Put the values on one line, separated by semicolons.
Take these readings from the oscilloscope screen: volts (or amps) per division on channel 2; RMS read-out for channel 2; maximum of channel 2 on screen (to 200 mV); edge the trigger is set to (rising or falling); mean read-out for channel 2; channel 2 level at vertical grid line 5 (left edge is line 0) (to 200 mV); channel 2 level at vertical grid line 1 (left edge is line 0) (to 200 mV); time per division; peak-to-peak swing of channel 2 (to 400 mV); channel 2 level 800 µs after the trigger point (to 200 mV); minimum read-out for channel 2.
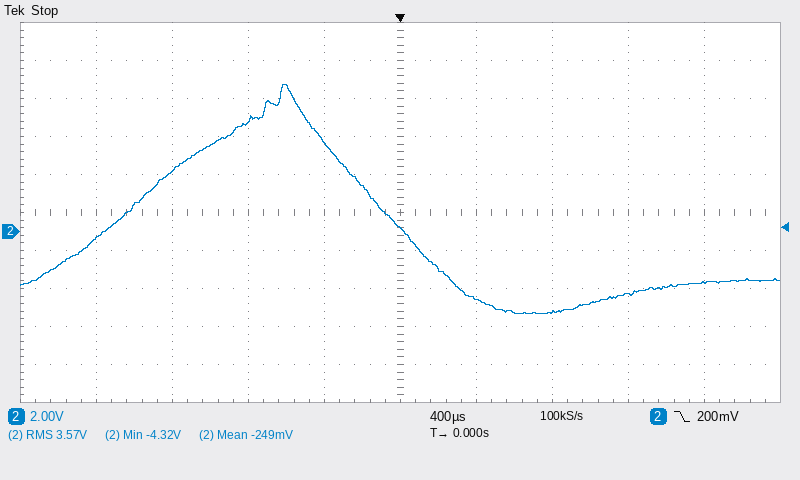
2 V; 3.57 V; 7.8 V; falling; -249 mV; 200 mV; -400 mV; 400 µs; 12.0 V; -4.2 V; -4.32 V
